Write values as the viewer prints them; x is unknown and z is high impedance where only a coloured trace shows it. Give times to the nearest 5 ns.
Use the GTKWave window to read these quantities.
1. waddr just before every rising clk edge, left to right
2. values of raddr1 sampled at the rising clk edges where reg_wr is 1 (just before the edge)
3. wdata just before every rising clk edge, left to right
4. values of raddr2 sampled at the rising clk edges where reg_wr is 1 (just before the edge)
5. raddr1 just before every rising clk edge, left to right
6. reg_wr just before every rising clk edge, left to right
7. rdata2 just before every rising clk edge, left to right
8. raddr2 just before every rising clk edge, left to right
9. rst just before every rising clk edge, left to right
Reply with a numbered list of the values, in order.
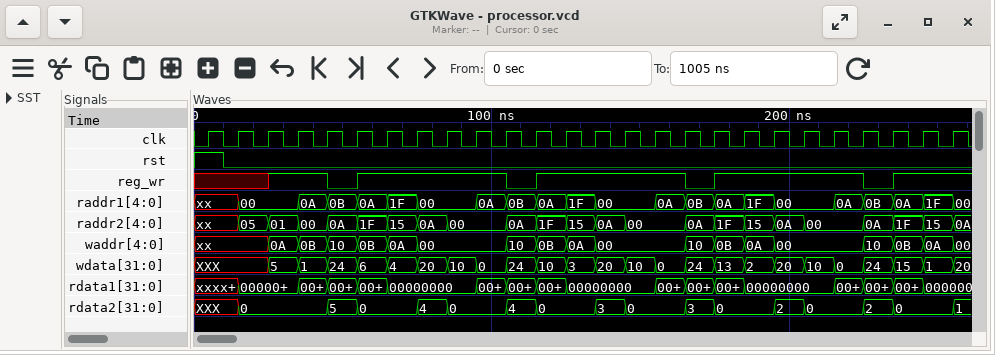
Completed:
1. xx, xx, xx, 0A, 0B, 10, 0B, 0A, 00, 00, 00, 10, 0B, 0A, 00, 00, 00, 10, 0B, 0A, 00, 00, 00, 10, 0B, 0A
2. 00, 0A, 0A, 1F, 00, 00, 0A, 0A, 1F, 00, 00, 0A, 0A, 1F, 00, 00, 0A, 0A, 1F
3. XXX, XXX, XXX, 5, 1, 24, 6, 4, 20, 10, 0, 24, 10, 3, 20, 10, 0, 24, 13, 2, 20, 10, 0, 24, 15, 1
4. 01, 00, 1F, 15, 0A, 00, 00, 1F, 15, 0A, 00, 00, 1F, 15, 0A, 00, 00, 1F, 15
5. xx, xx, 00, 00, 0A, 0B, 0A, 1F, 00, 00, 0A, 0B, 0A, 1F, 00, 00, 0A, 0B, 0A, 1F, 00, 00, 0A, 0B, 0A, 1F
6. x x x 1 1 0 1 1 1 1 1 0 1 1 1 1 1 0 1 1 1 1 1 0 1 1
7. XXX, XXX, 0, 0, 0, 5, 0, 0, 4, 0, 0, 4, 0, 0, 3, 0, 0, 3, 0, 0, 2, 0, 0, 2, 0, 0
8. xx, xx, 05, 01, 00, 0A, 1F, 15, 0A, 00, 00, 0A, 1F, 15, 0A, 00, 00, 0A, 1F, 15, 0A, 00, 00, 0A, 1F, 15
9. 1 0 0 0 0 0 0 0 0 0 0 0 0 0 0 0 0 0 0 0 0 0 0 0 0 0
